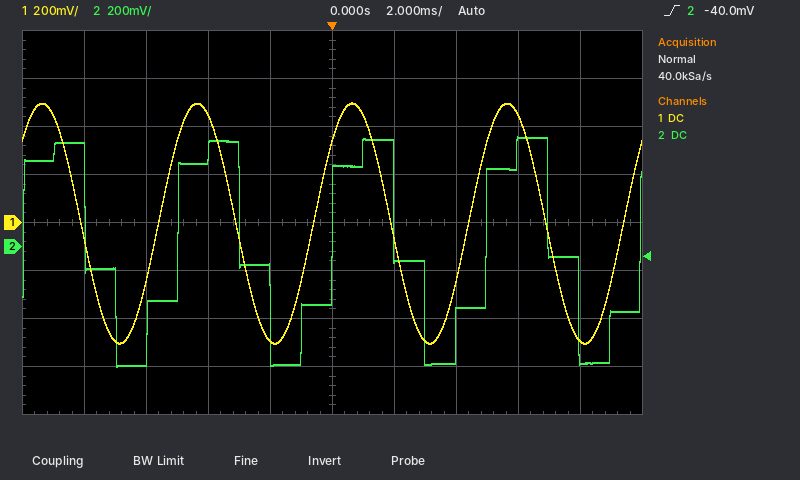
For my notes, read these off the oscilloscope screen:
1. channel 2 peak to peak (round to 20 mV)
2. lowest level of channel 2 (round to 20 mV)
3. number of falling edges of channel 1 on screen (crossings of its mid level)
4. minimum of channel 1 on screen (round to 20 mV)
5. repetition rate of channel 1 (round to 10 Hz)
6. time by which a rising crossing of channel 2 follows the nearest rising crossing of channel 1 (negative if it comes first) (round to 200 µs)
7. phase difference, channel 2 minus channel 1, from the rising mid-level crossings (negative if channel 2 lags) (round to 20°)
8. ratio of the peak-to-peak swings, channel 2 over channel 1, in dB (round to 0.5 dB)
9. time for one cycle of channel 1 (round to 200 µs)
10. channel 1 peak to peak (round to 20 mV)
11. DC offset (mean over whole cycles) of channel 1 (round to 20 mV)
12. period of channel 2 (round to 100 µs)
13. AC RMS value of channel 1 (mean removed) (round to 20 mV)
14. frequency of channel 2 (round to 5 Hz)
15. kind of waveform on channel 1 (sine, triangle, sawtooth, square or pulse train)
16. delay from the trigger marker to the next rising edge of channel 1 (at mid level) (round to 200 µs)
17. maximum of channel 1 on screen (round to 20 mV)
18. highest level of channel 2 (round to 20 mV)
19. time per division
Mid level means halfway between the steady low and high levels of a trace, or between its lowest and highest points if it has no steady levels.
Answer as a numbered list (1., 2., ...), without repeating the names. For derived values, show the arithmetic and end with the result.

1. 460 mV − (-500 mV) = 960 mV
2. -500 mV
3. 4
4. -500 mV
5. 1 / 5.0 ms ≈ 200 Hz
6. +600 µs
7. −360° × (+600 µs) / 5.0 ms ≈ -43.2°, so -40° to the nearest 20°
8. 20 log10(960 mV / 1.00 V) ≈ -0.355 dB, so -0.5 dB to the nearest 0.5 dB
9. 5.0 ms
10. 500 mV − (-500 mV) = 1.00 V
11. (500 mV + (-500 mV)) / 2 ≈ 0 mV
12. 5.0 ms
13. 1.00 V / (2√2) ≈ 354 mV, so 360 mV to the nearest 20 mV
14. 1 / 5.0 ms ≈ 200 Hz
15. sine
16. 4.4 ms
17. 500 mV
18. 460 mV
19. 2 ms
